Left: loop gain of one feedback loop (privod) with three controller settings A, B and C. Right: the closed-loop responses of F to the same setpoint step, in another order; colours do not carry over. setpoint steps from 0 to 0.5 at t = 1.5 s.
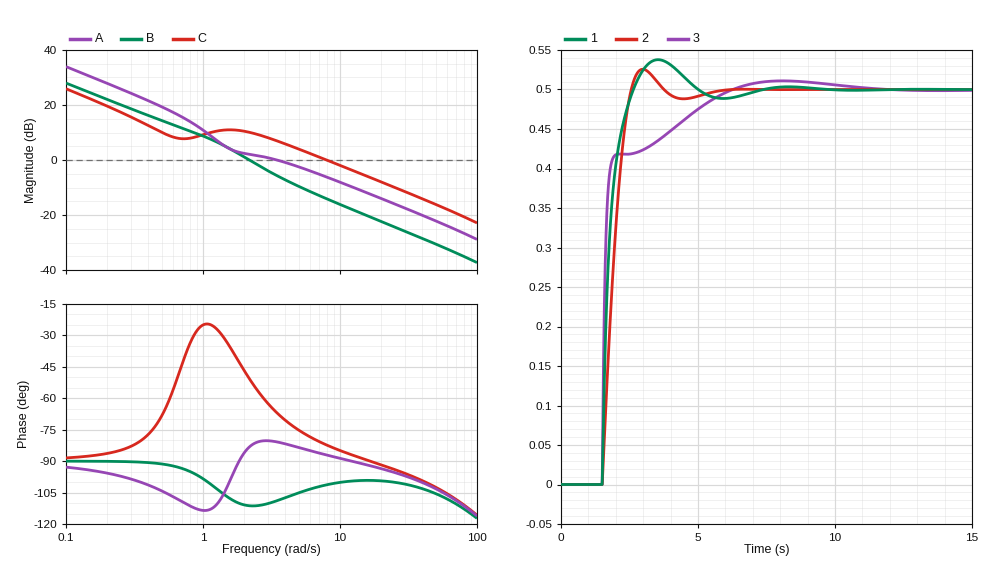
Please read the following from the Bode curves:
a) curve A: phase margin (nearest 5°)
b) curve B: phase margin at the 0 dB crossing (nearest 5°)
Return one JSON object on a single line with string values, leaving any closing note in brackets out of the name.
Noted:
{"curve A: phase margin": "100°", "curve B: phase margin at the 0 dB crossing": "70°"}
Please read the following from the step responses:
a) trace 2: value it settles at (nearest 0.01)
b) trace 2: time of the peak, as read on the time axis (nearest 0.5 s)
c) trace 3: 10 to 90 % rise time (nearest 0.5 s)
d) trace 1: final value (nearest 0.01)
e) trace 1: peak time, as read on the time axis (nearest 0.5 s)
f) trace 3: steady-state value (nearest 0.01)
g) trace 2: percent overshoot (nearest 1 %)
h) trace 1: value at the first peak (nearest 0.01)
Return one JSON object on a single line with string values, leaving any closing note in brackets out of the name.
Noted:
{"trace 2: value it settles at": "0.50", "trace 2: time of the peak, as read on the time axis": "3.0 s", "trace 3: 10 to 90 % rise time": "2.5 s", "trace 1: final value": "0.50", "trace 1: peak time, as read on the time axis": "3.5 s", "trace 3: steady-state value": "0.50", "trace 2: percent overshoot": "5 %", "trace 1: value at the first peak": "0.54"}
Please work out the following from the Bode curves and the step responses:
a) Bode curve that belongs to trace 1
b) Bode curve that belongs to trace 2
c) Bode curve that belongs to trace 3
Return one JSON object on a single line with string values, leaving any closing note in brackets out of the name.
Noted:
{"Bode curve that belongs to trace 1": "A", "Bode curve that belongs to trace 2": "B", "Bode curve that belongs to trace 3": "C"}
